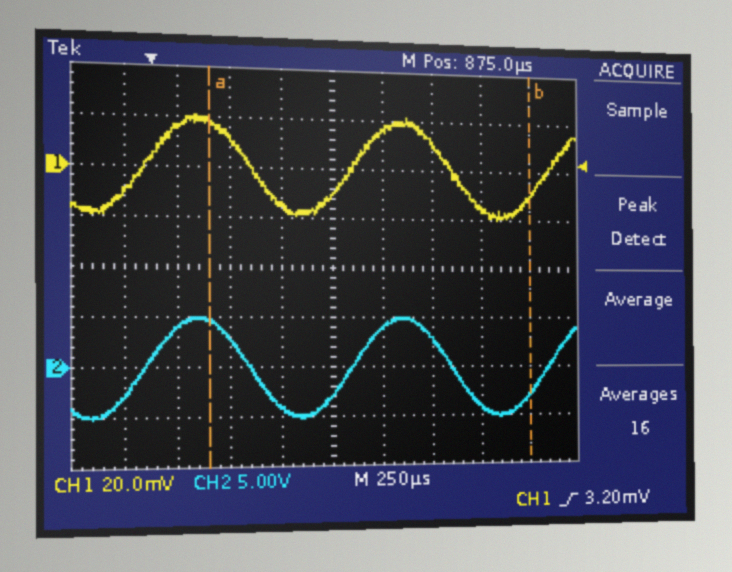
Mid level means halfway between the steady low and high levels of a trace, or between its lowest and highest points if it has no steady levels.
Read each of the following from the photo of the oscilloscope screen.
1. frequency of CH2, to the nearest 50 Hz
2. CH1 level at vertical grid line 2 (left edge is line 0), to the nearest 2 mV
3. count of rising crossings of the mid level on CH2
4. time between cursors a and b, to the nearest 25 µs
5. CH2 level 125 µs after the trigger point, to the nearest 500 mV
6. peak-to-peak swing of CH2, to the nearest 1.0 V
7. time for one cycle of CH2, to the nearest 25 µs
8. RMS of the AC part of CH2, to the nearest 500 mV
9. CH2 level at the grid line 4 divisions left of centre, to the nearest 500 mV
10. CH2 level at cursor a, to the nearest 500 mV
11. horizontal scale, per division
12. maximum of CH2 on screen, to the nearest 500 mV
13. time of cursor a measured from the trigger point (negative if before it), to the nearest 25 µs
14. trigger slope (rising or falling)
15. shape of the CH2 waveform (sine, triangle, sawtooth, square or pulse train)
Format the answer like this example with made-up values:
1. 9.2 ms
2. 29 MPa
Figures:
1. 1.00 kHz
2. 16 mV
3. 3
4. 1.600 ms
5. 4.0 V
6. 10.0 V
7. 1.000 ms
8. 3.5 V
9. -3.0 V
10. 4.5 V
11. 250 µs
12. 5.0 V
13. +275 µs
14. rising
15. sine
